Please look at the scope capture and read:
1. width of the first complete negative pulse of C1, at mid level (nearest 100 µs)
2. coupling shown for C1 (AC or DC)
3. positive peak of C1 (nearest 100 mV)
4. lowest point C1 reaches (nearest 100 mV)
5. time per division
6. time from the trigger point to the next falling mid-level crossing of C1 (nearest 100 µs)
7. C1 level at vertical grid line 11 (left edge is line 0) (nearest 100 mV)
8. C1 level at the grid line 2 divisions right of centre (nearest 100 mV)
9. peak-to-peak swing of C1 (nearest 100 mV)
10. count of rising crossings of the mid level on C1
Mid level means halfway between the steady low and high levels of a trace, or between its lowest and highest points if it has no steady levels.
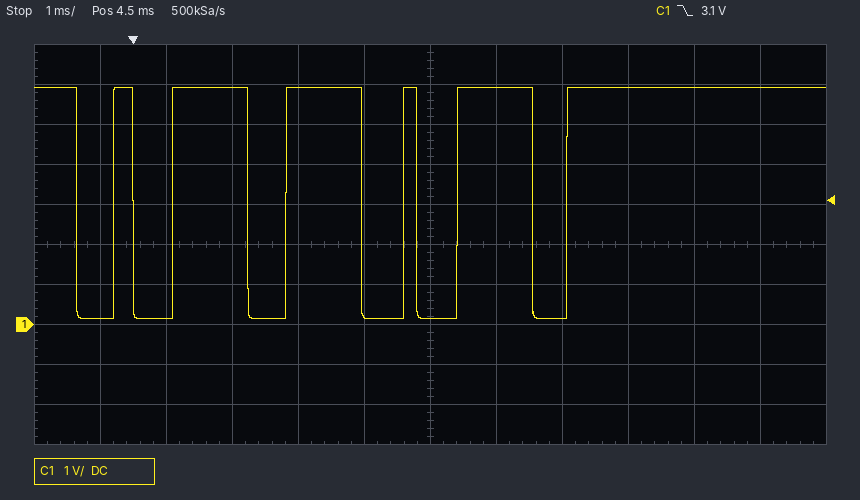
600 µs
DC
5.9 V
100 mV
1 ms
1.7 ms
5.9 V
100 mV
5.8 V
6
